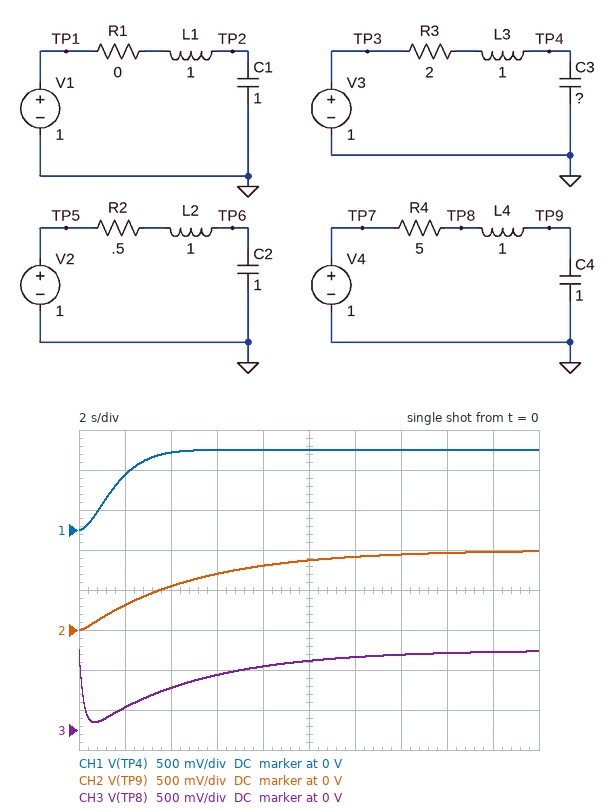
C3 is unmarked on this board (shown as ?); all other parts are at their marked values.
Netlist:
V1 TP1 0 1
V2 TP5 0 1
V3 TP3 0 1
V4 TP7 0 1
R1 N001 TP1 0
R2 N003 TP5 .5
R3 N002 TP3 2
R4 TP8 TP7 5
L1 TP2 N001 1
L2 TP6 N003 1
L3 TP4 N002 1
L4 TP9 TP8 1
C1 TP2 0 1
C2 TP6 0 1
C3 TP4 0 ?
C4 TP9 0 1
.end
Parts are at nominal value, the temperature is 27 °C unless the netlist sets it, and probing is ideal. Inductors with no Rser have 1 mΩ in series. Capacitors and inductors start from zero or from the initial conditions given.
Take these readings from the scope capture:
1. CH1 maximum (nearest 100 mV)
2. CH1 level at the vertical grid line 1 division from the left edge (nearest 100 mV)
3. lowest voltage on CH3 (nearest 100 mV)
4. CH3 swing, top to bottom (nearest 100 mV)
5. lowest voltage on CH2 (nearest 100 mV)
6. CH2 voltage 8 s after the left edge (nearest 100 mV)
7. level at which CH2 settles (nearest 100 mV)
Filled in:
1.0 V
700 mV
100 mV
900 mV
0 V
800 mV
1.0 V
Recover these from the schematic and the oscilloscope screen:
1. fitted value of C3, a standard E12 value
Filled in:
820 mF
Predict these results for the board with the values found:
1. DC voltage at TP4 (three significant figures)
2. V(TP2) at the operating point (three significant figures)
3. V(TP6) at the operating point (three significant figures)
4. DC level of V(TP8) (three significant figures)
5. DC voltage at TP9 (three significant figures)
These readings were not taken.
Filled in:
1.00 V
1.00 V
1.00 V
1.00 V
1.00 V
